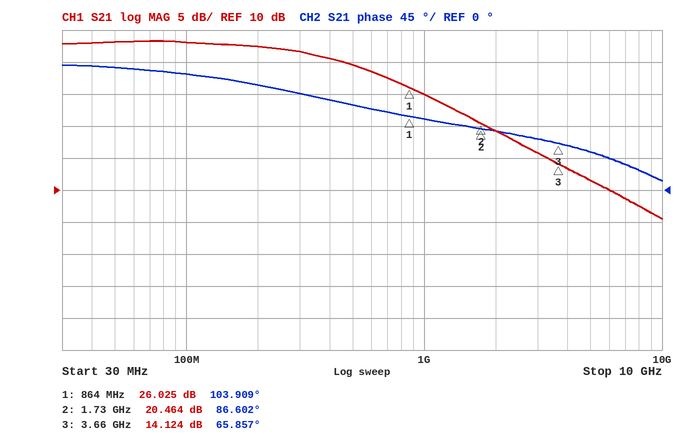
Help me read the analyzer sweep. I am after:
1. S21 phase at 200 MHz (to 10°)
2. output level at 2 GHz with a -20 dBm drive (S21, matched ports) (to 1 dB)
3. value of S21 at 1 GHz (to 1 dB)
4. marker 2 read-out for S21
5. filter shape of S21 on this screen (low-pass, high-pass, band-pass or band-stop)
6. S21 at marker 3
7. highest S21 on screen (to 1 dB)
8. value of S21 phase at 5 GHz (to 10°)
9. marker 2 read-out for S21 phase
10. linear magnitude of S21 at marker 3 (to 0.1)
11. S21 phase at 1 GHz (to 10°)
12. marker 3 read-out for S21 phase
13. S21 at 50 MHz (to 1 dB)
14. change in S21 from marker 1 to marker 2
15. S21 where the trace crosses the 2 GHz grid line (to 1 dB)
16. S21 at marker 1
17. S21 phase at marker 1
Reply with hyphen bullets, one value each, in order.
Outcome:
- 150°
- -1 dBm
- 25 dB
- 20.464 dB
- low-pass
- 14.124 dB
- 33 dB
- 50°
- 86.602°
- 5.1
- 100°
- 65.857°
- 33 dB
- -5.561 dB
- 19 dB
- 26.025 dB
- 103.909°
